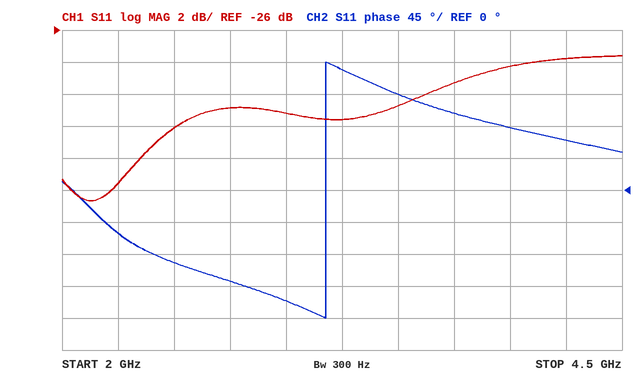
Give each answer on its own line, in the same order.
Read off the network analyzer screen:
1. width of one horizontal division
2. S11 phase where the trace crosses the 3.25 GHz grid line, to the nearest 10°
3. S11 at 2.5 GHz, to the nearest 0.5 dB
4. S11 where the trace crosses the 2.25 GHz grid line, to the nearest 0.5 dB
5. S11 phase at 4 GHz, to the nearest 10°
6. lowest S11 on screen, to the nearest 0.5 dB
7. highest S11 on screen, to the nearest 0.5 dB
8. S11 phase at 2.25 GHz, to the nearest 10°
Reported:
250 MHz
170°
-32.0 dB
-35.5 dB
90°
-36.5 dB
-27.5 dB
-60°
